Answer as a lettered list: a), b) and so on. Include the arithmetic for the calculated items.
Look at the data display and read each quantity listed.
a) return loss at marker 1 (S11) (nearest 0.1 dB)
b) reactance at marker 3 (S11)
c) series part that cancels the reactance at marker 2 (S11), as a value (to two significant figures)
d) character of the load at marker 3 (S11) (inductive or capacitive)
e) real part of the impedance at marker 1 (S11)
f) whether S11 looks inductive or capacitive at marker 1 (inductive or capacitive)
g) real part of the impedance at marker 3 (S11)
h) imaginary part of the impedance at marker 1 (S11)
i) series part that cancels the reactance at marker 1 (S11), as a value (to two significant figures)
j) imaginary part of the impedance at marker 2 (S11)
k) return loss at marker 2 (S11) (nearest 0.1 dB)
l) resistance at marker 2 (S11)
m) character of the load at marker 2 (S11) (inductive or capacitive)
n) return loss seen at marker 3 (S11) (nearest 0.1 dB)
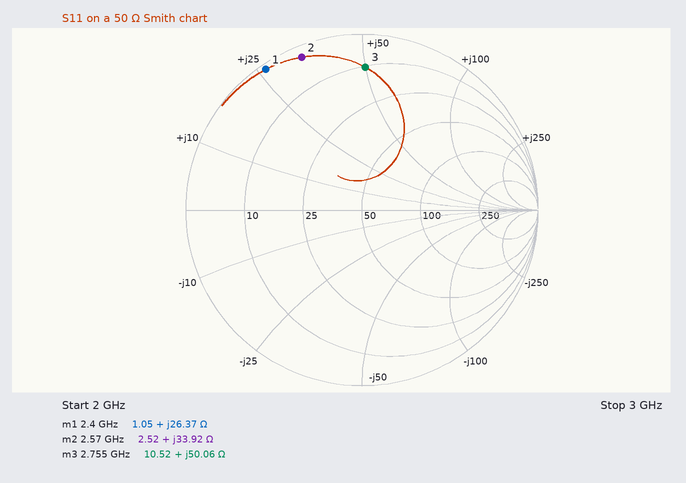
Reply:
a) 0.3 dB
b) +50.06 Ω
c) C = 1/(2π × 2.57 GHz × 33.92 Ω) ≈ 1.8 pF
d) inductive
e) 1.05 Ω
f) inductive
g) 10.52 Ω
h) +26.37 Ω
i) C = 1/(2π × 2.4 GHz × 26.37 Ω) ≈ 2.5 pF
j) +33.92 Ω
k) 0.6 dB
l) 2.52 Ω
m) inductive
n) 1.8 dB
